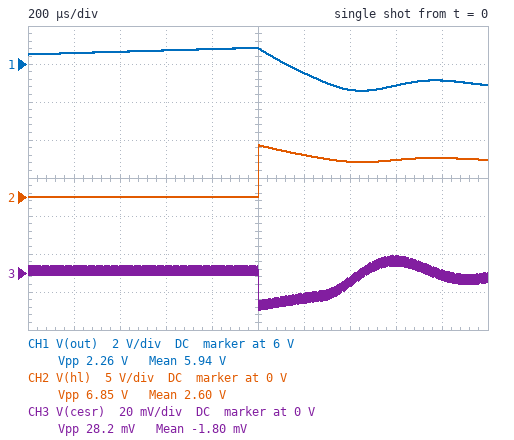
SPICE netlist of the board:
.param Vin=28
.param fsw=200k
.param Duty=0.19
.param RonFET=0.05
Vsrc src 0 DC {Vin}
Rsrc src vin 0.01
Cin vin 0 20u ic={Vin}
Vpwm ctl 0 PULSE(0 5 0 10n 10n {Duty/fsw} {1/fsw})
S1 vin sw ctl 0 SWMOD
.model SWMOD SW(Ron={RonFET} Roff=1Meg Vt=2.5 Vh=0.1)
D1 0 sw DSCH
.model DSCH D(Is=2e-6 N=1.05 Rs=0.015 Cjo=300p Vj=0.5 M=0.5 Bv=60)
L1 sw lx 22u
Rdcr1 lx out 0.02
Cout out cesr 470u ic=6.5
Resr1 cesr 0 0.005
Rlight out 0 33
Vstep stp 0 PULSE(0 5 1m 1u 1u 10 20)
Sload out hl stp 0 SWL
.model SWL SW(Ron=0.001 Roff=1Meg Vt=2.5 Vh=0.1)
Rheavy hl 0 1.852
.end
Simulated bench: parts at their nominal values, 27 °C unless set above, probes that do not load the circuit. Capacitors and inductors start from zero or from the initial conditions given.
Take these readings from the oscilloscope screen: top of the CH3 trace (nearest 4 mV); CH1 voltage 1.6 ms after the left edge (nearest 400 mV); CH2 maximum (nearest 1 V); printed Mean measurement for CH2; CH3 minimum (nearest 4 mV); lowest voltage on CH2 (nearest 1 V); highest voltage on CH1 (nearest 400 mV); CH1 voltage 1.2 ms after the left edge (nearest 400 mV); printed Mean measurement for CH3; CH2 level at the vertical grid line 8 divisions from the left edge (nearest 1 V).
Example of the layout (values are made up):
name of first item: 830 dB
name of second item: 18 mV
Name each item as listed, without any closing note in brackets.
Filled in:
top of the CH3 trace: 8 mV
CH1 voltage 1.6 ms after the left edge: 4.8 V
CH2 maximum: 7 V
printed Mean measurement for CH2: 2.60 V
CH3 minimum: -20 mV
lowest voltage on CH2: 0 V
highest voltage on CH1: 6.8 V
CH1 voltage 1.2 ms after the left edge: 5.6 V
printed Mean measurement for CH3: -1.80 mV
CH2 level at the vertical grid line 8 divisions from the left edge: 5 V
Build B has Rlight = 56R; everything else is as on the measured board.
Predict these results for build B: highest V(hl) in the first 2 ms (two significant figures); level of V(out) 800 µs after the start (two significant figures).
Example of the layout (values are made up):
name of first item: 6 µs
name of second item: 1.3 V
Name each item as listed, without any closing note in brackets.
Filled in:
highest V(hl) in the first 2 ms: 7.0 V
level of V(out) 800 µs after the start: 6.9 V
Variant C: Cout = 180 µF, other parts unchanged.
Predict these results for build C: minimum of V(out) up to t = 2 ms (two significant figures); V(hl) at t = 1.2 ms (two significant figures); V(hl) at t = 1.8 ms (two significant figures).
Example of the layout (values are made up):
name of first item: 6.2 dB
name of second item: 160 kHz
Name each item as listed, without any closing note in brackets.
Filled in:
minimum of V(out) up to t = 2 ms: 4.3 V
V(hl) at t = 1.2 ms: 4.4 V
V(hl) at t = 1.8 ms: 5.0 V
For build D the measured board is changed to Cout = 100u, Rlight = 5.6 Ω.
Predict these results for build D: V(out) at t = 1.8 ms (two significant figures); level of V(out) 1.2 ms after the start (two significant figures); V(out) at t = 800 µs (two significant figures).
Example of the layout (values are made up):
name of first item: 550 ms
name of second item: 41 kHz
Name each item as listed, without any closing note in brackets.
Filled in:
V(out) at t = 1.8 ms: 4.9 V
level of V(out) 1.2 ms after the start: 5.3 V
V(out) at t = 800 µs: 5.1 V
